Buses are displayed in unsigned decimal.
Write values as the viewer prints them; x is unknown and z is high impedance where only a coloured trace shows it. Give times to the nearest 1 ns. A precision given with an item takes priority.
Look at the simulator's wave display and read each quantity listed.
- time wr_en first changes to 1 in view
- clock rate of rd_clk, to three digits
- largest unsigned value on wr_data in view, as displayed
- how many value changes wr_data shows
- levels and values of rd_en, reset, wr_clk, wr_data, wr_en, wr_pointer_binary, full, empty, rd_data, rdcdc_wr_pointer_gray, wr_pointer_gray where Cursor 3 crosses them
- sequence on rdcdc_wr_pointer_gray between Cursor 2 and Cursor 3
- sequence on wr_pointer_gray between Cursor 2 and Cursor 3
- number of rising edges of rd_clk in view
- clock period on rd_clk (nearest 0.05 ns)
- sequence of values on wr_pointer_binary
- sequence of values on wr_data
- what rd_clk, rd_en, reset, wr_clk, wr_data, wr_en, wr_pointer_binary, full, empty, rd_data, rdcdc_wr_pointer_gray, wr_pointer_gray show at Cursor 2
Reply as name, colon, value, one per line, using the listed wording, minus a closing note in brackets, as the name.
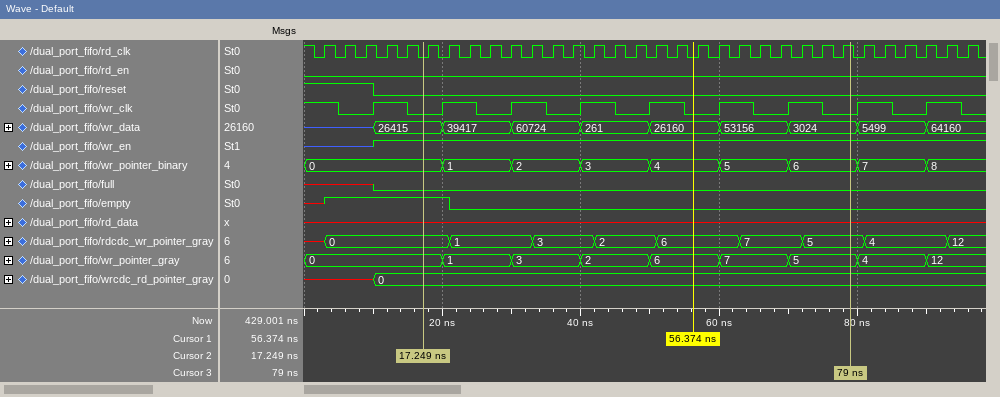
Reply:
time wr_en first changes to 1 in view: 10 ns
clock rate of rd_clk, to three digits: 333 MHz
largest unsigned value on wr_data in view, as displayed: 64160
how many value changes wr_data shows: 9
levels and values of rd_en, reset, wr_clk, wr_data, wr_en, wr_pointer_binary, full, empty, rd_data, rdcdc_wr_pointer_gray, wr_pointer_gray where Cursor 3 crosses them: rd_en=0, reset=0, wr_clk=0, wr_data=3024, wr_en=1, wr_pointer_binary=6, full=0, empty=0, rd_data=x, rdcdc_wr_pointer_gray=5, wr_pointer_gray=5
sequence on rdcdc_wr_pointer_gray between Cursor 2 and Cursor 3: 0, 1, 3, 2, 6, 7, 5
sequence on wr_pointer_gray between Cursor 2 and Cursor 3: 0, 1, 3, 2, 6, 7, 5
number of rising edges of rd_clk in view: 32
clock period on rd_clk: 3 ns
sequence of values on wr_pointer_binary: 0, 1, 2, 3, 4, 5, 6, 7, 8
sequence of values on wr_data: z, 26415, 39417, 60724, 261, 26160, 53156, 3024, 5499, 64160
what rd_clk, rd_en, reset, wr_clk, wr_data, wr_en, wr_pointer_binary, full, empty, rd_data, rdcdc_wr_pointer_gray, wr_pointer_gray show at Cursor 2: rd_clk=0, rd_en=0, reset=0, wr_clk=0, wr_data=26415, wr_en=1, wr_pointer_binary=0, full=0, empty=1, rd_data=x, rdcdc_wr_pointer_gray=0, wr_pointer_gray=0
